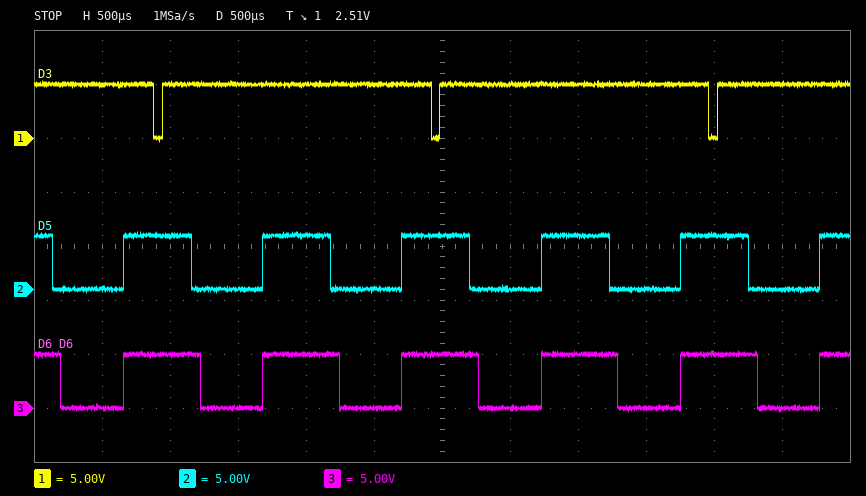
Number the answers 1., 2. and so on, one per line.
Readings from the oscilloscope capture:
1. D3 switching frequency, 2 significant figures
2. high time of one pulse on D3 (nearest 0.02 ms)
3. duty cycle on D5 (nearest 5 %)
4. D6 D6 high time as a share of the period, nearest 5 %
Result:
1. 490 Hz
2. 1.98 ms
3. 50 %
4. 55 %
